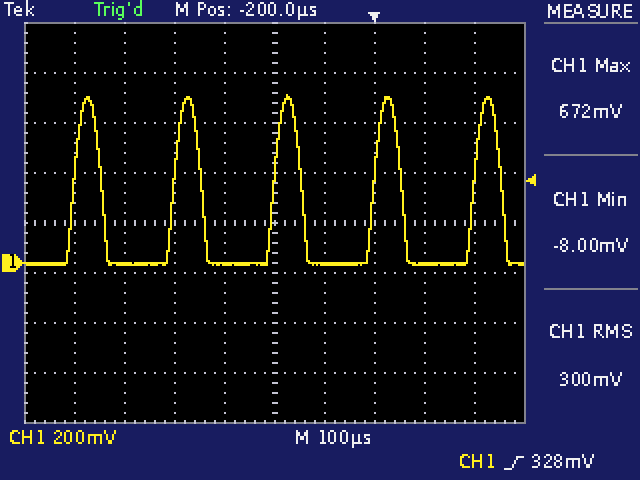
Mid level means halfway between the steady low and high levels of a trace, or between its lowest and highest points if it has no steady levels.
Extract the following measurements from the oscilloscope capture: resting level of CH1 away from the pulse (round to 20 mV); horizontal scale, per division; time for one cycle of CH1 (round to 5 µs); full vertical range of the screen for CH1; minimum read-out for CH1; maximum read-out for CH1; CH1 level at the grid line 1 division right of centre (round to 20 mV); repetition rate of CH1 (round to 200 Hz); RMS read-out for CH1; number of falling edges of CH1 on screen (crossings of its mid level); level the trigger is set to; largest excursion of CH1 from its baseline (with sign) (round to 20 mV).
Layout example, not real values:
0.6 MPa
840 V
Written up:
0 mV
100 µs
200 µs
1.6 V
-8.00 mV
672 mV
0 mV
5.0 kHz
300 mV
5
328 mV
+680 mV
